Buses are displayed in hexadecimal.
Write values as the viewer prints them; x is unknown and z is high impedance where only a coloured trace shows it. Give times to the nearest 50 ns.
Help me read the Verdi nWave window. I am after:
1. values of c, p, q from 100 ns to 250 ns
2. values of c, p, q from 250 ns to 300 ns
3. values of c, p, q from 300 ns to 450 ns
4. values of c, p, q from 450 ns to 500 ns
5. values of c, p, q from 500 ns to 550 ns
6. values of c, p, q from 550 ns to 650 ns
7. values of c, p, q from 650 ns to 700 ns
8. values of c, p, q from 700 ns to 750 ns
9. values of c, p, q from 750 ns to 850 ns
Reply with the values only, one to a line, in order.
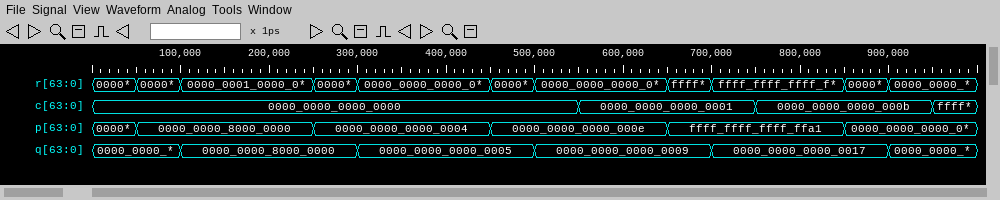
c=0000_0000_0000_0000, p=0000_0000_8000_0000, q=0000_0000_8000_0000
c=0000_0000_0000_0000, p=0000_0000_0000_0004, q=0000_0000_8000_0000
c=0000_0000_0000_0000, p=0000_0000_0000_0004, q=0000_0000_0000_0005
c=0000_0000_0000_0000, p=0000_0000_0000_000e, q=0000_0000_0000_0005
c=0000_0000_0000_0000, p=0000_0000_0000_000e, q=0000_0000_0000_0009
c=0000_0000_0000_0001, p=0000_0000_0000_000e, q=0000_0000_0000_0009
c=0000_0000_0000_0001, p=ffff_ffff_ffff_ffa1, q=0000_0000_0000_0009
c=0000_0000_0000_0001, p=ffff_ffff_ffff_ffa1, q=0000_0000_0000_0017
c=0000_0000_0000_000b, p=ffff_ffff_ffff_ffa1, q=0000_0000_0000_0017
